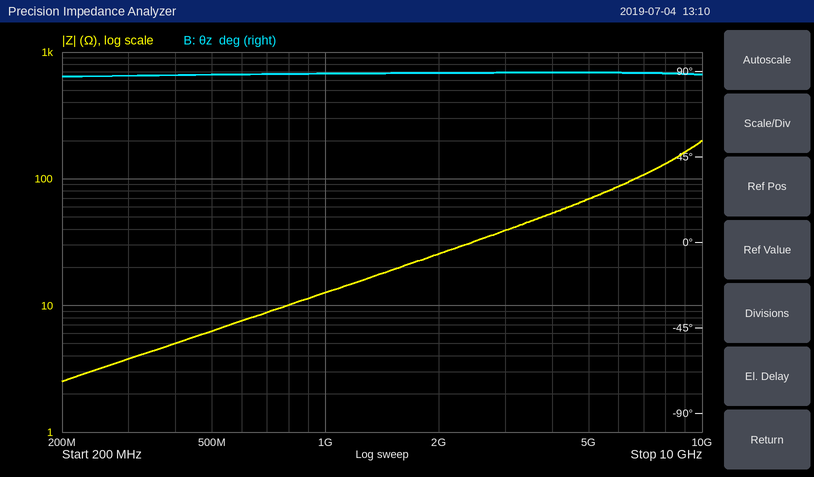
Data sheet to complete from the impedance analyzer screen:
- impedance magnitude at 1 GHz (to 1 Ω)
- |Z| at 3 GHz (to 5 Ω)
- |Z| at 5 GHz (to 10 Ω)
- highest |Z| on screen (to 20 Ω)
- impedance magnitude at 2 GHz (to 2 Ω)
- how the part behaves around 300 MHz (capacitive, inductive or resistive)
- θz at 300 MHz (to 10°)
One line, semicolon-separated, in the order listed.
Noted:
13 Ω; 40 Ω; 70 Ω; 200 Ω; 26 Ω; inductive; 90°
